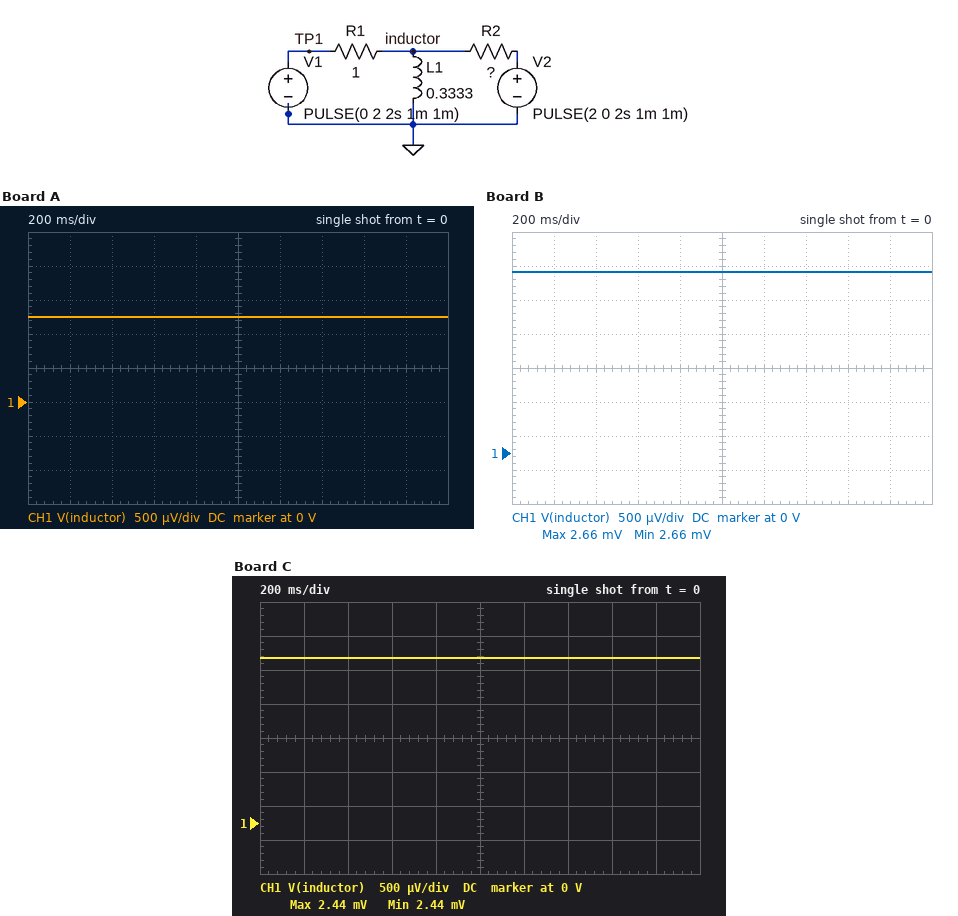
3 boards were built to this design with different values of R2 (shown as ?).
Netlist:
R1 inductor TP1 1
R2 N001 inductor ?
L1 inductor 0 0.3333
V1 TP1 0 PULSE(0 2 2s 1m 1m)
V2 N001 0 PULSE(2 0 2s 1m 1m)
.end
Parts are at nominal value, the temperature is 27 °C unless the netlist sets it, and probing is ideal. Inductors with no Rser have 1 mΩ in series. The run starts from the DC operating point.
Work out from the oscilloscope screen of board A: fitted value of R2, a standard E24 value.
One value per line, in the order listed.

1.6 Ω
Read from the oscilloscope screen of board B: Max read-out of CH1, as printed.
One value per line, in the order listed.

2.66 mV
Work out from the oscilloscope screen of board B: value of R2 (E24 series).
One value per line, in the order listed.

0.75 Ω
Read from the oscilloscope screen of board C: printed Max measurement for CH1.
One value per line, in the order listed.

2.44 mV
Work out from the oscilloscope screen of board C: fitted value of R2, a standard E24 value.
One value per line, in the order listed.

0.82 Ω
